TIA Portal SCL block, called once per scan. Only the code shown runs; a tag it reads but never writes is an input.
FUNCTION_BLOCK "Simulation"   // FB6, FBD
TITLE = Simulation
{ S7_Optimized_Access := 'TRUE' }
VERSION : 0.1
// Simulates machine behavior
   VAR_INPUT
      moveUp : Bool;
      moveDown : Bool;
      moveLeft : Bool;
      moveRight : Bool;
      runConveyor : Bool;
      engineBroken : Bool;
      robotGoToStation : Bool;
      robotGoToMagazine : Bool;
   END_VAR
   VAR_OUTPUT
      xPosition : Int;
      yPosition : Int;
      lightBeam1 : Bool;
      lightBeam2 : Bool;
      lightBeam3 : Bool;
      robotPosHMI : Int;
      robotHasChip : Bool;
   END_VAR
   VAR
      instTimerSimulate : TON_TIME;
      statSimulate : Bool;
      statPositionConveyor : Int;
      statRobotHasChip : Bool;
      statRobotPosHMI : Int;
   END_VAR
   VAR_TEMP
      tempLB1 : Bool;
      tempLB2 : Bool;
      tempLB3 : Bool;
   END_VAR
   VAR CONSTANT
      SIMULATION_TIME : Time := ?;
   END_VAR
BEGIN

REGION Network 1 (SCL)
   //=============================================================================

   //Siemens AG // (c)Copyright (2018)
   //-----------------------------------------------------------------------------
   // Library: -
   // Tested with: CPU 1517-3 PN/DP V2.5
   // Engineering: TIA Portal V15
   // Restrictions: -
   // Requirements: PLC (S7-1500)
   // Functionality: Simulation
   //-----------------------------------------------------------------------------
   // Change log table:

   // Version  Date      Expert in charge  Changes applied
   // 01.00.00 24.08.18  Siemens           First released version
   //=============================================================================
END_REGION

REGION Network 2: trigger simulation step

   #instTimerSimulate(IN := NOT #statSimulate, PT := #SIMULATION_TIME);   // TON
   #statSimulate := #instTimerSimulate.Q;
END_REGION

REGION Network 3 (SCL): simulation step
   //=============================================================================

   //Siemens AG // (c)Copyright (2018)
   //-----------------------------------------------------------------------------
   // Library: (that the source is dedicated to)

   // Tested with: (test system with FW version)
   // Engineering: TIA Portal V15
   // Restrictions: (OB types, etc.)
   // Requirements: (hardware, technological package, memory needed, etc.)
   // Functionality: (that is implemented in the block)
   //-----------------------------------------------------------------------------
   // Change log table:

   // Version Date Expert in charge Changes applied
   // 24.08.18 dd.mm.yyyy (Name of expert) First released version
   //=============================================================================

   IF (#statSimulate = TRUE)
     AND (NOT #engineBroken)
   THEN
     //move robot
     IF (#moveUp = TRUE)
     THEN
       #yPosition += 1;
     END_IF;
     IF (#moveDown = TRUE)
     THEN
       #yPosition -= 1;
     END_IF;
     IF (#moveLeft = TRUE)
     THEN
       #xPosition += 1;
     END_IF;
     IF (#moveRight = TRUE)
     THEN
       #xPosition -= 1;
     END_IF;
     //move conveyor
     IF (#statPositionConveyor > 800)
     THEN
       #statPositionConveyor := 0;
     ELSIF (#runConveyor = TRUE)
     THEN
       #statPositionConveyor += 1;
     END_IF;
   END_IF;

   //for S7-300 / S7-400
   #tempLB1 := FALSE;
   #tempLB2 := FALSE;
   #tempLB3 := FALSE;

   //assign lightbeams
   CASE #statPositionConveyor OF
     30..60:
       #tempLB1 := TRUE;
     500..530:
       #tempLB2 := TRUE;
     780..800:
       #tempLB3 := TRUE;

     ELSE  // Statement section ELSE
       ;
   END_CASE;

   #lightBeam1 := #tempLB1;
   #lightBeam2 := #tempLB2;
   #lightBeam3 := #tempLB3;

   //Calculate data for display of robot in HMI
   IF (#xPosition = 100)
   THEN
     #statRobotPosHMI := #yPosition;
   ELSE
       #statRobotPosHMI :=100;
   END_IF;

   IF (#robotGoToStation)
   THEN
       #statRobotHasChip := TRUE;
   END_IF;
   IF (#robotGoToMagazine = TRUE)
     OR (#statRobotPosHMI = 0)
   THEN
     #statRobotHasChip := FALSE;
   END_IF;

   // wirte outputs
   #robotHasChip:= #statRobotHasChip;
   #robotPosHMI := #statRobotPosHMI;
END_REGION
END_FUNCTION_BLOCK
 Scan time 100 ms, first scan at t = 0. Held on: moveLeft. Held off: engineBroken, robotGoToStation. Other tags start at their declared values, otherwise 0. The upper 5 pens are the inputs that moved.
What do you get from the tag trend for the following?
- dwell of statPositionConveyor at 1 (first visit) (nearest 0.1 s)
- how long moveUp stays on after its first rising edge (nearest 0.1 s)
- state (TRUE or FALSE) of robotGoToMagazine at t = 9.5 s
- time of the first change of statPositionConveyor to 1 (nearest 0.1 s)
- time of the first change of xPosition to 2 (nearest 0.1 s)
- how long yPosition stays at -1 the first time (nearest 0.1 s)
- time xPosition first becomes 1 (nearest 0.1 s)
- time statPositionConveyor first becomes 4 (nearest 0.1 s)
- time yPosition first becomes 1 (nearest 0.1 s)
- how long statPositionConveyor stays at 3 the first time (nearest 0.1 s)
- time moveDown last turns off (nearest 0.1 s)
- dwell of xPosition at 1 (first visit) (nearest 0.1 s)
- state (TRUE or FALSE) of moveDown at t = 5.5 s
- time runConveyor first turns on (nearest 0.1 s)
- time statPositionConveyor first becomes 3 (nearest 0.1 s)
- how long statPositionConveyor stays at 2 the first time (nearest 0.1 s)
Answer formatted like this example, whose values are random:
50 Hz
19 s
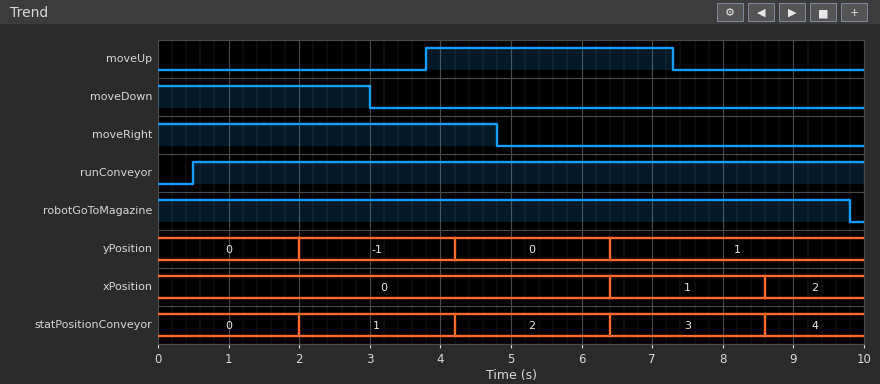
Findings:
2.2 s
3.5 s
TRUE
2.0 s
8.6 s
2.2 s
6.4 s
8.6 s
6.4 s
2.2 s
3.0 s
2.2 s
FALSE
0.5 s
6.4 s
2.2 s
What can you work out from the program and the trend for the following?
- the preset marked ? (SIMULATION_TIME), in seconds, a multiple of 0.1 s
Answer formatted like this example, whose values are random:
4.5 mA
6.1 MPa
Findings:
2.0 s
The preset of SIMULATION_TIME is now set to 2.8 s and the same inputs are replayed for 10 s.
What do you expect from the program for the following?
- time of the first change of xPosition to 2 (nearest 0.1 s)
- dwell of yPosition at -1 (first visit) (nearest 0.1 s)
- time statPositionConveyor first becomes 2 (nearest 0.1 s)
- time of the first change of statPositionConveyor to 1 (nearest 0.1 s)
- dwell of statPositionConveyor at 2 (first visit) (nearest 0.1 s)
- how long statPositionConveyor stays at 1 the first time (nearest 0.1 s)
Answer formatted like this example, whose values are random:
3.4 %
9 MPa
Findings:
8.8 s
3.0 s
5.8 s
2.8 s
3.0 s
3.0 s
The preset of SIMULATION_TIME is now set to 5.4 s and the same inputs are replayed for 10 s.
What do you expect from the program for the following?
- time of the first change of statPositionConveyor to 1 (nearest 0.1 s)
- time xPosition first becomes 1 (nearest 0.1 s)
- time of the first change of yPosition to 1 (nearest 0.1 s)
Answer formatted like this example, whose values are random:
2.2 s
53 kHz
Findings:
5.4 s
5.4 s
5.4 s
